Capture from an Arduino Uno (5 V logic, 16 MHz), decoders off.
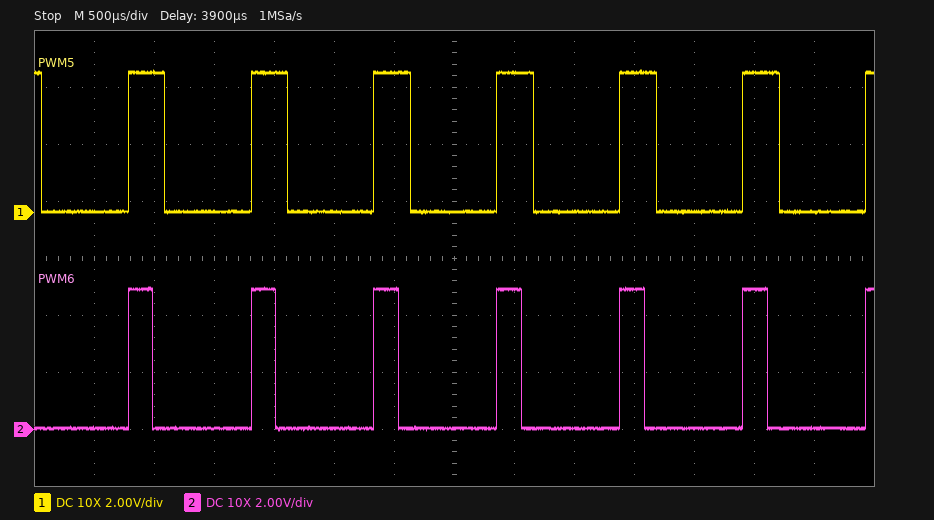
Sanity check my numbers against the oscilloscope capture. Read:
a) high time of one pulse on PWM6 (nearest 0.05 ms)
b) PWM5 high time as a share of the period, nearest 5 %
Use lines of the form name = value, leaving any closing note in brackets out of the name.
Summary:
high time of one pulse on PWM6 = 0.20 ms
PWM5 high time as a share of the period, nearest 5 % = 30 %
